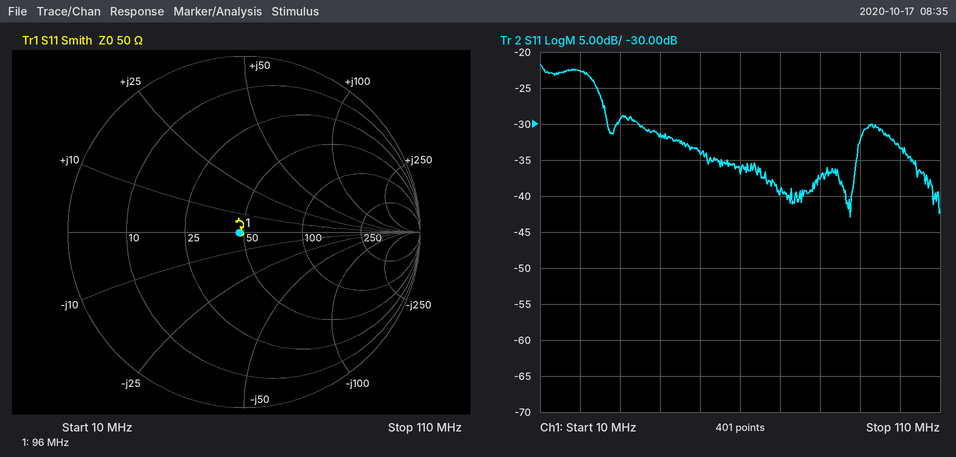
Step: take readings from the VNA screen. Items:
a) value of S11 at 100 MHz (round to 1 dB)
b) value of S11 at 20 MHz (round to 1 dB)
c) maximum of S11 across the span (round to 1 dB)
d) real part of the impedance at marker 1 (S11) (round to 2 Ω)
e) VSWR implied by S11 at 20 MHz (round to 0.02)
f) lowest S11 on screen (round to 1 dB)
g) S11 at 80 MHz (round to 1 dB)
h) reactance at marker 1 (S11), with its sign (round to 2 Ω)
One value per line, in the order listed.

-33 dB
-23 dB
-22 dB
48 Ω
1.16
-43 dB
-38 dB
0 Ω
